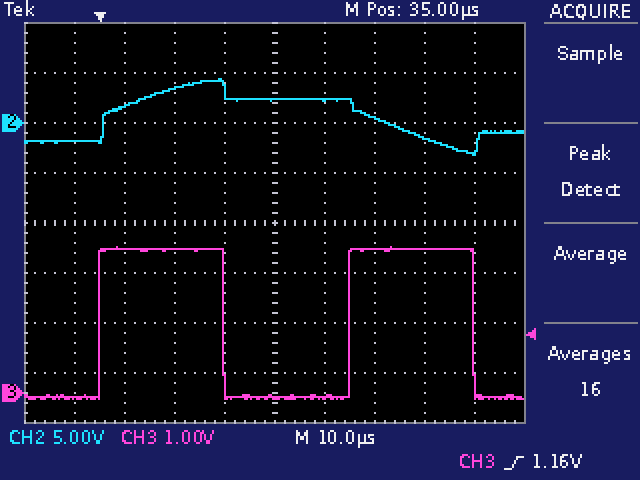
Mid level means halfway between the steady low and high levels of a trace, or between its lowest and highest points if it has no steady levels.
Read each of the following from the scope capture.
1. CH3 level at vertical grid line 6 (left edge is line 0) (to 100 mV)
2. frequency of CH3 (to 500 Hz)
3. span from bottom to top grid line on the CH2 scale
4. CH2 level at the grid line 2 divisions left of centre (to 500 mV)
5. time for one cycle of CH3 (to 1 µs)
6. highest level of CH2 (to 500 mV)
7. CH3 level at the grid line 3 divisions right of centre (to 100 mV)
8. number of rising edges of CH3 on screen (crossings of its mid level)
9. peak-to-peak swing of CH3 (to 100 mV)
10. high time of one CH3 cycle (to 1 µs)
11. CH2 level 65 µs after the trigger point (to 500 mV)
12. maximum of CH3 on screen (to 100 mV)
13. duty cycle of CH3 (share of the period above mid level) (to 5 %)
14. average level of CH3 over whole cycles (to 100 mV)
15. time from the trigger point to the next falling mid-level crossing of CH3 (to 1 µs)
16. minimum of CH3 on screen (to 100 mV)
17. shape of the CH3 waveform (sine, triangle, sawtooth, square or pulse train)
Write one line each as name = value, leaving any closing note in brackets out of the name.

CH3 level at vertical grid line 6 (left edge is line 0) = -100 mV
frequency of CH3 = 20.0 kHz
span from bottom to top grid line on the CH2 scale = 40 V
CH2 level at the grid line 2 divisions left of centre = 3.5 V
time for one cycle of CH3 = 50 µs
highest level of CH2 = 4.5 V
CH3 level at the grid line 3 divisions right of centre = 2.9 V
number of rising edges of CH3 on screen = 2
peak-to-peak swing of CH3 = 3.0 V
high time of one CH3 cycle = 25 µs
CH2 level 65 µs after the trigger point = -1.5 V
maximum of CH3 on screen = 2.9 V
duty cycle of CH3 (share of the period above mid level) = 50 %
average level of CH3 over whole cycles = 1.4 V
time from the trigger point to the next falling mid-level crossing of CH3 = 25 µs
minimum of CH3 on screen = -100 mV
shape of the CH3 waveform = square
